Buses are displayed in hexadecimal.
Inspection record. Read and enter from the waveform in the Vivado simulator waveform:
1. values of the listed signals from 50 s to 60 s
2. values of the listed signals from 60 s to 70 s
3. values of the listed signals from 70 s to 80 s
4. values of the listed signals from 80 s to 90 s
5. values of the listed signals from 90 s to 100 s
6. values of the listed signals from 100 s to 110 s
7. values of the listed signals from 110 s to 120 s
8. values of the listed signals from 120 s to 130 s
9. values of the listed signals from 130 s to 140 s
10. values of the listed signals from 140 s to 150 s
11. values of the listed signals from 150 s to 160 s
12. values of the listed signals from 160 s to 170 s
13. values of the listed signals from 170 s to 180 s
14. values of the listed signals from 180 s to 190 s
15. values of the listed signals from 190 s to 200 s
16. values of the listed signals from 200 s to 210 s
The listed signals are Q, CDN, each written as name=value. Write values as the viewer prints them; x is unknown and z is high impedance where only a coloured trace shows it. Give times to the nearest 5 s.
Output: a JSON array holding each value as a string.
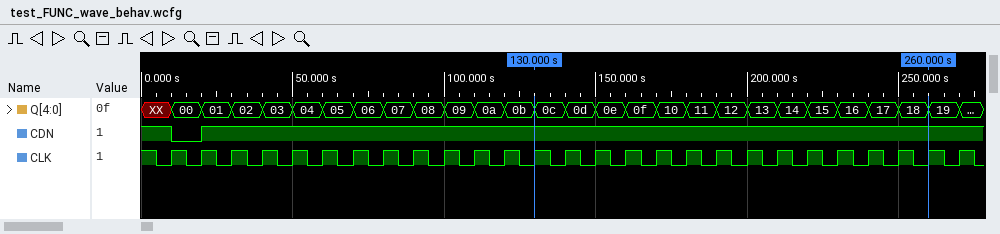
["Q=04, CDN=1", "Q=05, CDN=1", "Q=06, CDN=1", "Q=07, CDN=1", "Q=08, CDN=1", "Q=09, CDN=1", "Q=0a, CDN=1", "Q=0b, CDN=1", "Q=0c, CDN=1", "Q=0d, CDN=1", "Q=0e, CDN=1", "Q=0f, CDN=1", "Q=10, CDN=1", "Q=11, CDN=1", "Q=12, CDN=1", "Q=13, CDN=1"]
